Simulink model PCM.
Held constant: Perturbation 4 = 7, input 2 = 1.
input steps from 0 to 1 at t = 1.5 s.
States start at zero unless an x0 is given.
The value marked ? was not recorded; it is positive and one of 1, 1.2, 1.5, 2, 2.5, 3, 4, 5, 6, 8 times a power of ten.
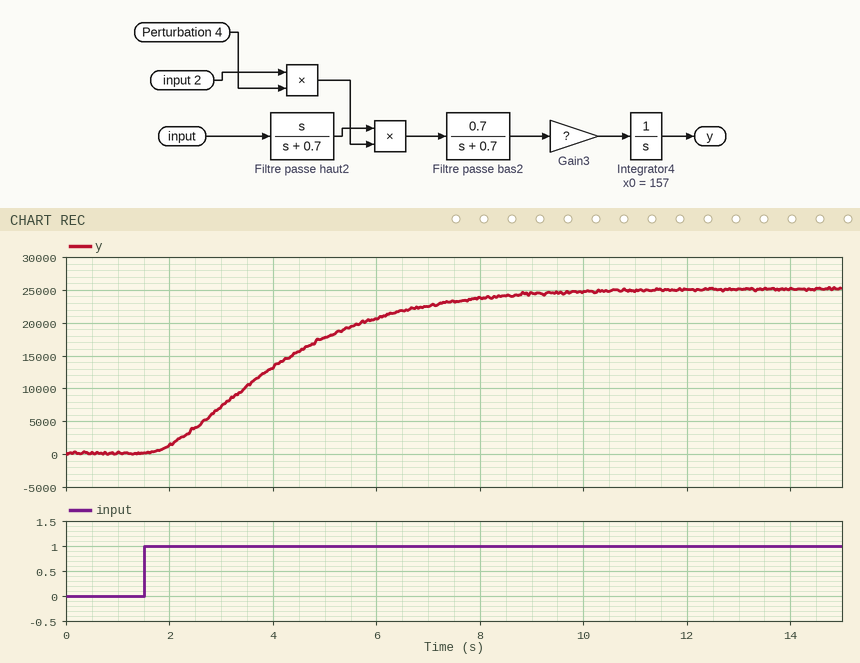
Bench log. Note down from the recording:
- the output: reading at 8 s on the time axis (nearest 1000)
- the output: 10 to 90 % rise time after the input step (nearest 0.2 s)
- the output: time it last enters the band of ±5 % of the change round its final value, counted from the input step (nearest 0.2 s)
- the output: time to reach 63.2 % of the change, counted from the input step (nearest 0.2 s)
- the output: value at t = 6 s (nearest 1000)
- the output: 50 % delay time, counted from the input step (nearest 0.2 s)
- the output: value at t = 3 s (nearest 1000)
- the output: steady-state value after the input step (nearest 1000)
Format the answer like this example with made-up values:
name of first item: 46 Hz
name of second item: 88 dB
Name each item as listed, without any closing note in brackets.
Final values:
the output: reading at 8 s on the time axis: 24000
the output: 10 to 90 % rise time after the input step: 4.8 s
the output: time it last enters the band of ±5 % of the change round its final value, counted from the input step: 6.8 s
the output: time to reach 63.2 % of the change, counted from the input step: 3.0 s
the output: value at t = 6 s: 21000
the output: 50 % delay time, counted from the input step: 2.4 s
the output: value at t = 3 s: 7000
the output: steady-state value after the input step: 25000
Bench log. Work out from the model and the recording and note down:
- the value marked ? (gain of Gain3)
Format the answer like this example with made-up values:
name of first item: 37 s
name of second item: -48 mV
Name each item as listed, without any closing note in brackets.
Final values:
the value marked ?: 2500
